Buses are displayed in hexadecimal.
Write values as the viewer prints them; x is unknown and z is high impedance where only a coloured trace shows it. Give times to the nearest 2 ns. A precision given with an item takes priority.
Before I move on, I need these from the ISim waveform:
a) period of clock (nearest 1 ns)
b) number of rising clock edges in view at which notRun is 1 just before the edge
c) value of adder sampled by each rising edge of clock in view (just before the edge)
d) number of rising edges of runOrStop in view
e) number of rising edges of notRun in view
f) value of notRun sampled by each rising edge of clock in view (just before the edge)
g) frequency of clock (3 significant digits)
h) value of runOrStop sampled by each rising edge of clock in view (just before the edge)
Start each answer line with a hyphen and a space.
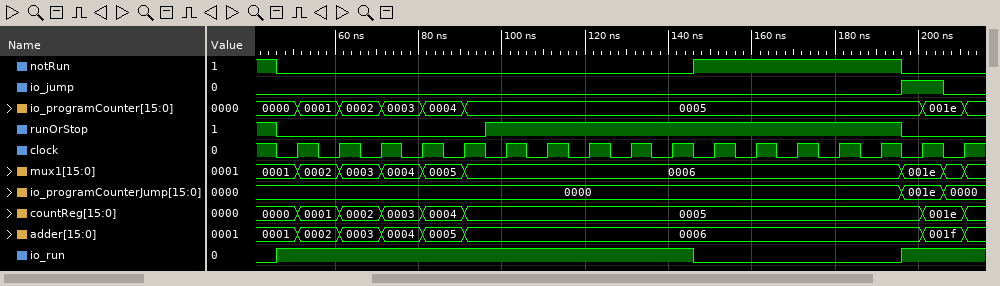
- 10 ns
- 5
- 0001, 0002, 0003, 0004, 0005, 0006, 0006, 0006, 0006, 0006, 0006, 0006, 0006, 0006, 0006, 0006, 001f
- 1
- 1
- 0 0 0 0 0 0 0 0 0 0 1 1 1 1 1 0 0
- 100 MHz
- 0 0 0 0 0 1 1 1 1 1 1 1 1 1 1 0 0
